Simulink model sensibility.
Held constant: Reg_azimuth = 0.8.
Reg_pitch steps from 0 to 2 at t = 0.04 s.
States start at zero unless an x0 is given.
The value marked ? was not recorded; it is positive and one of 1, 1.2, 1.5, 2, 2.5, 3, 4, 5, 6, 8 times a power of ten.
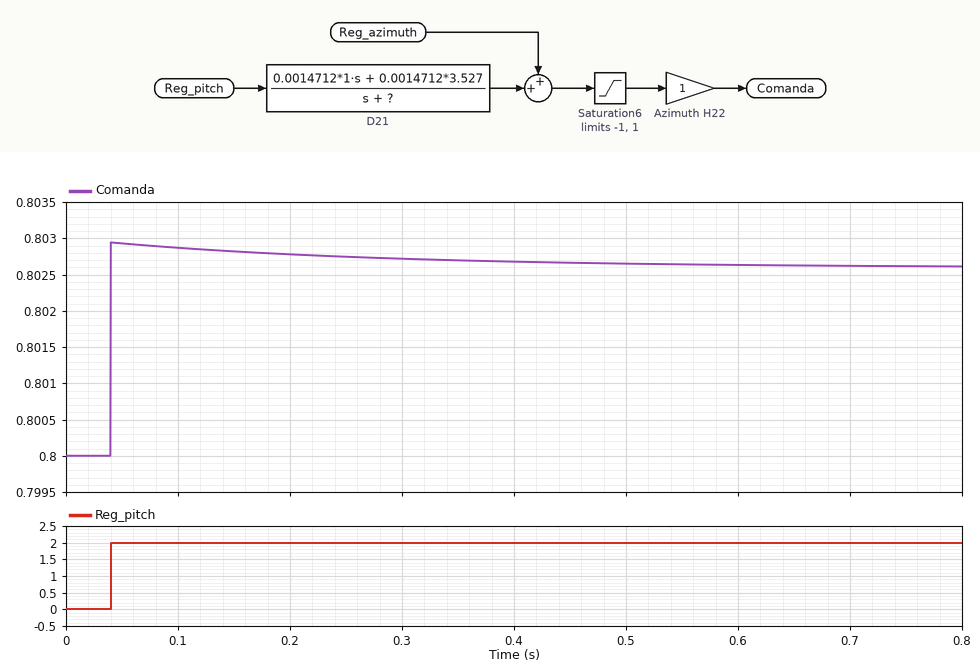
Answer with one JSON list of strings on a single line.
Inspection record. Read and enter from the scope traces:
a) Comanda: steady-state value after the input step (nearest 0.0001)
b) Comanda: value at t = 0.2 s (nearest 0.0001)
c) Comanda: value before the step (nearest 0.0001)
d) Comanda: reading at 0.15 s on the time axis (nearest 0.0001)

["0.8026", "0.8028", "0.8000", "0.8028"]
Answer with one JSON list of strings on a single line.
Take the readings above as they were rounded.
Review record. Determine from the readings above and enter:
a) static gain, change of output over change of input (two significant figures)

["0.0013"]
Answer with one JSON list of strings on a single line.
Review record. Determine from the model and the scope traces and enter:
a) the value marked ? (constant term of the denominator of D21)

["4"]
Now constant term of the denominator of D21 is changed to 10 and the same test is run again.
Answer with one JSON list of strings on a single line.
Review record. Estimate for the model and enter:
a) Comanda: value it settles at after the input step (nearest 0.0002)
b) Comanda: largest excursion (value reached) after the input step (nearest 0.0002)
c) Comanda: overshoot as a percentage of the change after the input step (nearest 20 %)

["0.8010", "0.8030", "180 %"]
